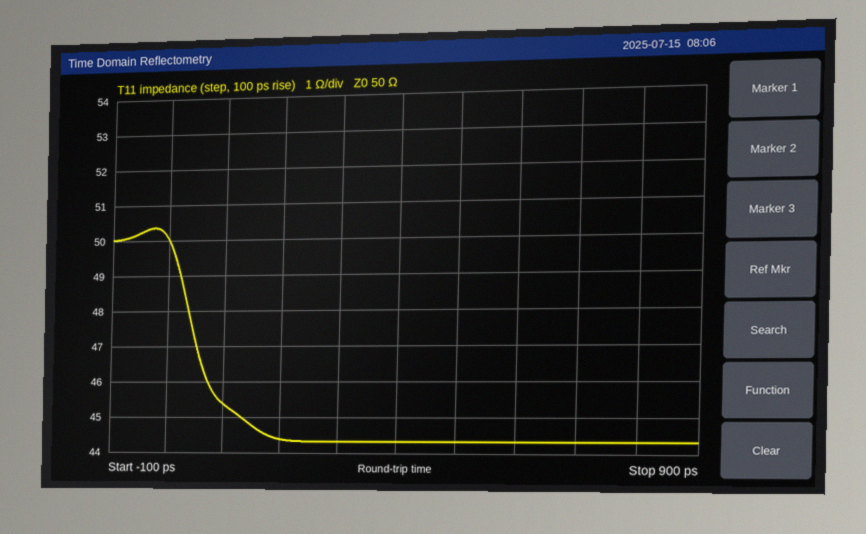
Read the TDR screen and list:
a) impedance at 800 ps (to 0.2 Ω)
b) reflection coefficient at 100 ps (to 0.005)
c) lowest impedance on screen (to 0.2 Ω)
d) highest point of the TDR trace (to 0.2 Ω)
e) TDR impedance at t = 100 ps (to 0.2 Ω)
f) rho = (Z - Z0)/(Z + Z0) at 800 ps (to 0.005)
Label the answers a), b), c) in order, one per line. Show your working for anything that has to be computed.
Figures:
a) 44.4 Ω
b) (45.4 − 50)/(45.4 + 50) ≈ -0.0482, so -0.050 to the nearest 0.005
c) 44.4 Ω
d) 50.4 Ω
e) 45.4 Ω
f) (44.4 − 50)/(44.4 + 50) ≈ -0.0593, so -0.060 to the nearest 0.005
